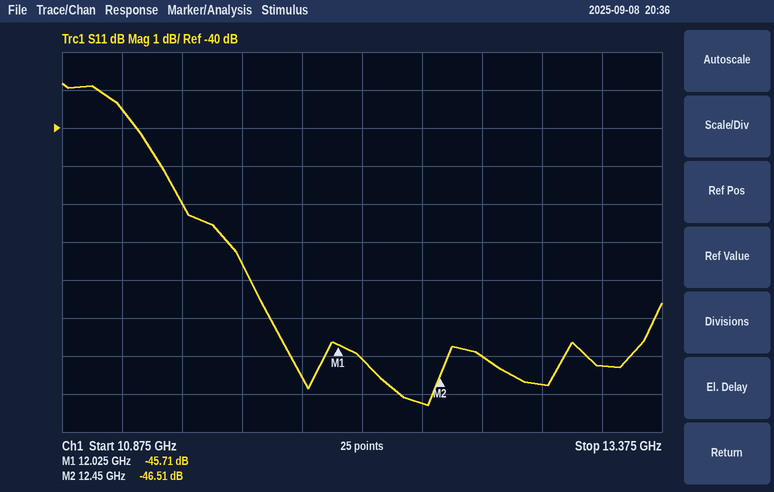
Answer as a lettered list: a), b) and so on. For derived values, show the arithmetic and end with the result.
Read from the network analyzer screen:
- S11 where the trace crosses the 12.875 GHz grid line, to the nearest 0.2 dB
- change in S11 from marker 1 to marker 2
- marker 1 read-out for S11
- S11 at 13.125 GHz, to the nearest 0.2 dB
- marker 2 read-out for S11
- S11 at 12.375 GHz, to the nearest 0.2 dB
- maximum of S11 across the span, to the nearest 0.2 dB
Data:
a) -46.8 dB
b) -46.51 − (-45.71) = -0.80 dB
c) -45.71 dB
d) -46.2 dB
e) -46.51 dB
f) -47.2 dB
g) -38.8 dB
